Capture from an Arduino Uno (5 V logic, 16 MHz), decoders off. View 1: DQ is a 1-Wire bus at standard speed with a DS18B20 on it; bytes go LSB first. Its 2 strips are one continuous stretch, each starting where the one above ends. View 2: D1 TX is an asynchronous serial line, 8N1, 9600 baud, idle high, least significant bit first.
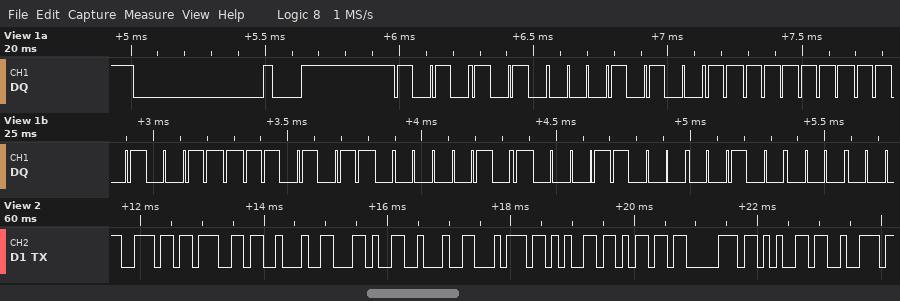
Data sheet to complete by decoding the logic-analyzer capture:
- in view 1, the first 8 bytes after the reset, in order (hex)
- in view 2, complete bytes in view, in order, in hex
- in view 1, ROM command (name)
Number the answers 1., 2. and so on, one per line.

1. 55 28 FF CB D7 A0 18 04
2. 0x6E 0x67 0x22 0x2C 0x22 0x74 0x65 0x6D 0x70 0x65 0x72
3. Match ROM
